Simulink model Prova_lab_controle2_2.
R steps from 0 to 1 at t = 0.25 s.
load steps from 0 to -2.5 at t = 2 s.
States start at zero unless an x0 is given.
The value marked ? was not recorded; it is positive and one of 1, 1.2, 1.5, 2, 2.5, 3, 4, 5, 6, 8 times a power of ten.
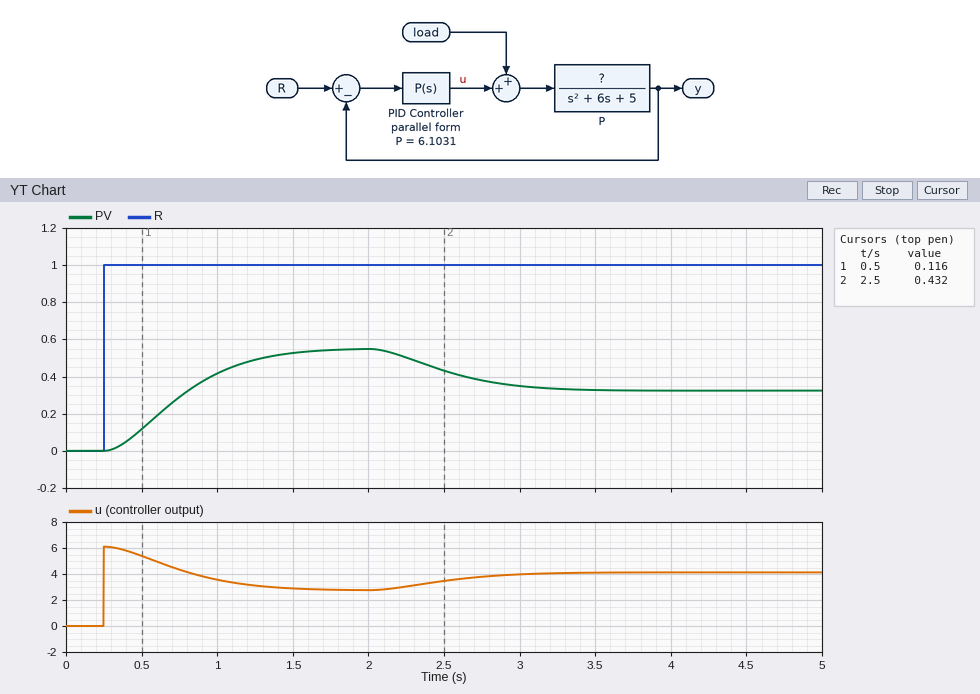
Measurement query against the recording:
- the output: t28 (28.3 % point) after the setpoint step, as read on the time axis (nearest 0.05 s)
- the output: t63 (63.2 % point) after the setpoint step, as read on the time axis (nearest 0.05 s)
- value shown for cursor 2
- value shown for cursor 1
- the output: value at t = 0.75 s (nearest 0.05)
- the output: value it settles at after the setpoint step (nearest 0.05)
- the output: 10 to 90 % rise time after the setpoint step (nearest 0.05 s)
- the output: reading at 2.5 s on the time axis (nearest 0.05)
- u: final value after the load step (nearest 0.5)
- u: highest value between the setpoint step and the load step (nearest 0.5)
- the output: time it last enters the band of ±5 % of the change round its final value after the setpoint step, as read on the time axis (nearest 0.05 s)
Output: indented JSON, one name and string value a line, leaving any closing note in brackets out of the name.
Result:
{
  "the output: t28 (28.3 % point) after the setpoint step, as read on the time axis": "0.55 s",
  "the output: t63 (63.2 % point) after the setpoint step, as read on the time axis": "0.85 s",
  "value shown for cursor 2": "0.432",
  "value shown for cursor 1": "0.116",
  "the output: value at t = 0.75 s": "0.30",
  "the output: value it settles at after the setpoint step": "0.55",
  "the output: 10 to 90 % rise time after the setpoint step": "0.85 s",
  "the output: reading at 2.5 s on the time axis": "0.45",
  "u: final value after the load step": "4.0",
  "u: highest value between the setpoint step and the load step": "6.0",
  "the output: time it last enters the band of ±5 % of the change round its final value after the setpoint step, as read on the time axis": "1.45 s"
}
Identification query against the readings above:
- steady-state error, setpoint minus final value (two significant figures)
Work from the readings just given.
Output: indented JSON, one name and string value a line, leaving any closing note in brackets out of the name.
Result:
{
  "steady-state error, setpoint minus final value": "0.45"
}
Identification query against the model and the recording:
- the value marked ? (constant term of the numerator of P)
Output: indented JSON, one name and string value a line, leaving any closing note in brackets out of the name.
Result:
{
  "the value marked ?": "1"
}
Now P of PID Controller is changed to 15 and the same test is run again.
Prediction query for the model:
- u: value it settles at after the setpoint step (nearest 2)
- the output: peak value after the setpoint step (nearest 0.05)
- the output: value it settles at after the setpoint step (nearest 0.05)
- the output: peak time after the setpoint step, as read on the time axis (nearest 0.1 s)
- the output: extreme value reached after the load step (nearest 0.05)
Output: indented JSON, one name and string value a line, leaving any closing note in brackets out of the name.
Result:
{
  "u: value it settles at after the setpoint step": "4",
  "the output: peak value after the setpoint step": "0.80",
  "the output: value it settles at after the setpoint step": "0.75",
  "the output: peak time after the setpoint step, as read on the time axis": "1.2 s",
  "the output: extreme value reached after the load step": "0.60"
}
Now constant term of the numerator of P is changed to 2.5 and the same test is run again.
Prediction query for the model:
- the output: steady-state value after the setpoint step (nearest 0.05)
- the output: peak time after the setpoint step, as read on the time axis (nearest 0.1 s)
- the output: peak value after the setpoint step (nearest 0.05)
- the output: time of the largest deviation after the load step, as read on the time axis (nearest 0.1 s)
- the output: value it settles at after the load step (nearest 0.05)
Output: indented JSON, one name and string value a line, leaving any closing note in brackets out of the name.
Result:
{
  "the output: steady-state value after the setpoint step": "0.75",
  "the output: peak time after the setpoint step, as read on the time axis": "1.2 s",
  "the output: peak value after the setpoint step": "0.80",
  "the output: time of the largest deviation after the load step, as read on the time axis": "2.9 s",
  "the output: value it settles at after the load step": "0.45"
}
